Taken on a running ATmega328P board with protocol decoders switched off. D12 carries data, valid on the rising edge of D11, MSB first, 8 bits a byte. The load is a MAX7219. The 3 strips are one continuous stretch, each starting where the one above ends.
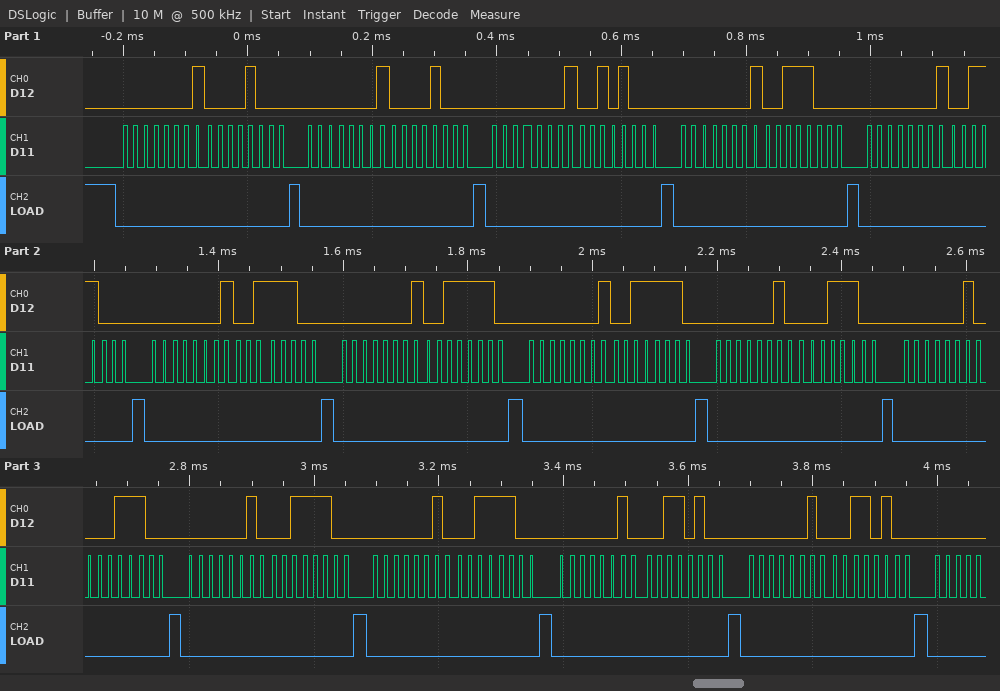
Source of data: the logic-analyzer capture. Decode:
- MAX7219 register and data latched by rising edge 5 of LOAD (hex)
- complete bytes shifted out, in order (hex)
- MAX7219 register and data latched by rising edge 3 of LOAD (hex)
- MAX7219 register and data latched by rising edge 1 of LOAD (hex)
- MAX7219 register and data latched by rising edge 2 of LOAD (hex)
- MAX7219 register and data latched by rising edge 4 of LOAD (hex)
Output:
register 0x1, data 0x38
01 08 01 08 01 28 01 38 01 38 01 3C 01 3E 01 3E 02 1C 02 1C 02 3C 02 3C 02 34 02 34
register 0x1, data 0x28
register 0x1, data 0x08
register 0x1, data 0x08
register 0x1, data 0x38
